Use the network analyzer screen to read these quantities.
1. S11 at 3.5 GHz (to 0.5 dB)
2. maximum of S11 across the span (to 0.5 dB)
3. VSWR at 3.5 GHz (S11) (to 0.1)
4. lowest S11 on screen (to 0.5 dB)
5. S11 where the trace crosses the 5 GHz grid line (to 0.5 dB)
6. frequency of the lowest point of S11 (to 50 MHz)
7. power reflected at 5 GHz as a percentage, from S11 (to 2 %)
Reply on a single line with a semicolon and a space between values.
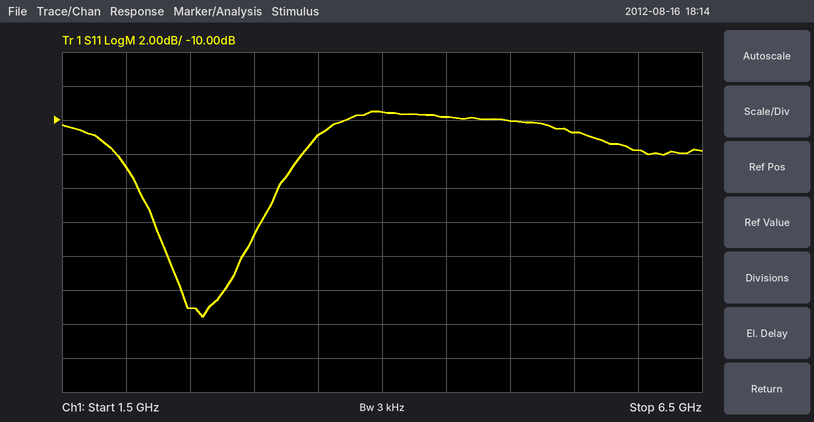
-11.0 dB; -9.5 dB; 1.8; -21.5 dB; -10.0 dB; 2.60 GHz; 10 %
